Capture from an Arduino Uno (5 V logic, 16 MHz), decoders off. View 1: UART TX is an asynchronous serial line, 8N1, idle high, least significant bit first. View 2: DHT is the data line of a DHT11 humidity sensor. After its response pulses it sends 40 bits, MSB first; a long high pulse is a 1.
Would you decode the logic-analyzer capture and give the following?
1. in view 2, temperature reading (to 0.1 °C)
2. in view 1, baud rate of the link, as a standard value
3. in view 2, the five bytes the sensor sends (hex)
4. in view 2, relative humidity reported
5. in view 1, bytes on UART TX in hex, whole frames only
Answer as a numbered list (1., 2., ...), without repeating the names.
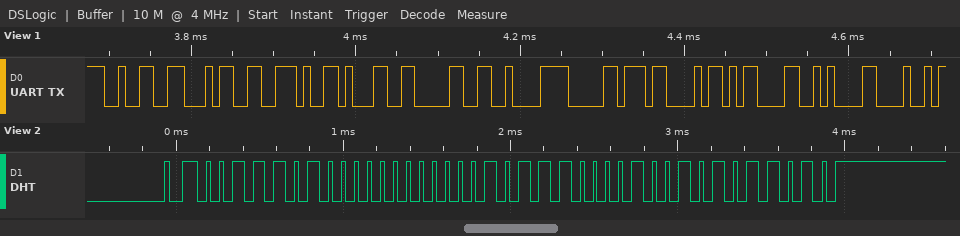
1. 23.9 °C
2. 115200 baud
3. 3A 00 17 09 5A
4. 58 %
5. 32 34 2E 31 30 C2 B0 43 0D 0A 48
